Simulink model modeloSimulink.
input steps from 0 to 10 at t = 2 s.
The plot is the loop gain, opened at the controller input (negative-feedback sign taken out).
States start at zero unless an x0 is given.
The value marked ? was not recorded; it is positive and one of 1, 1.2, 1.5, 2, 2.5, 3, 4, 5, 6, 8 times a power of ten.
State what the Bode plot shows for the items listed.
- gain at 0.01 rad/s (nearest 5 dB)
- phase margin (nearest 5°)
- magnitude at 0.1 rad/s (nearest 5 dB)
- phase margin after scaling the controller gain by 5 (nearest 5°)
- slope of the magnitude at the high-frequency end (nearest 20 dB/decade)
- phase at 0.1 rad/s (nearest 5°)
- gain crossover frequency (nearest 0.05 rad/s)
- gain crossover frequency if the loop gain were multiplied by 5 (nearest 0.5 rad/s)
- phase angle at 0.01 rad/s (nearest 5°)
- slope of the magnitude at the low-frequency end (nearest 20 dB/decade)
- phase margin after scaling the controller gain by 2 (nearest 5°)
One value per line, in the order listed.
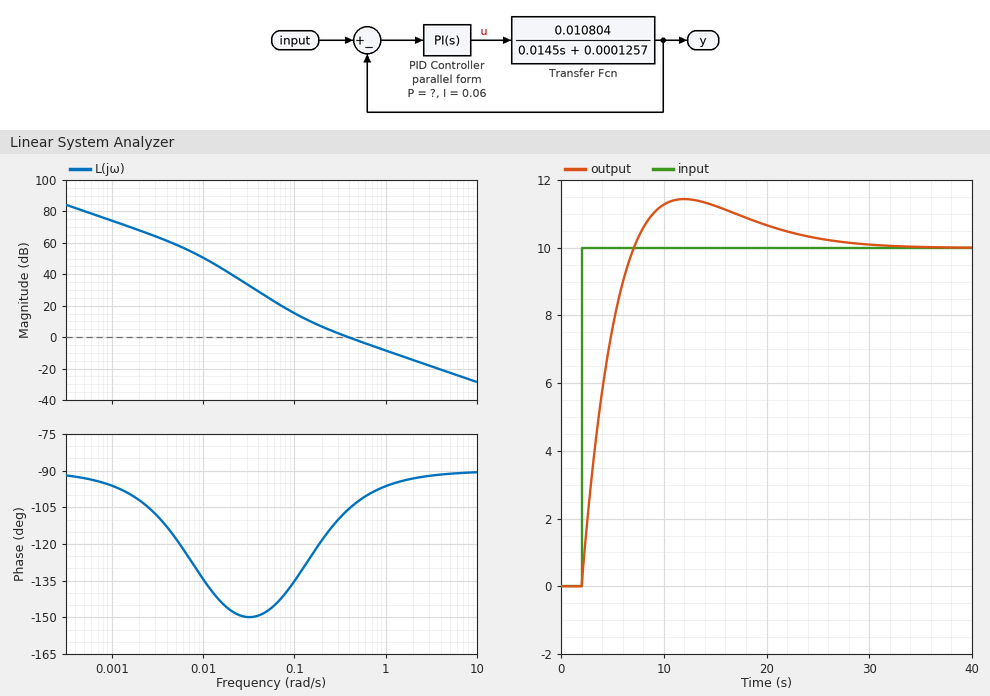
50 dB
75°
15 dB
85°
-20 dB/decade
-135°
0.40 rad/s
2.0 rad/s
-135°
-20 dB/decade
80°
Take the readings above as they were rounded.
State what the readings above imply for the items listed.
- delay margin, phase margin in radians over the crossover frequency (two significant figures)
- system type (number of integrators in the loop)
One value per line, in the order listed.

3.3 s
1
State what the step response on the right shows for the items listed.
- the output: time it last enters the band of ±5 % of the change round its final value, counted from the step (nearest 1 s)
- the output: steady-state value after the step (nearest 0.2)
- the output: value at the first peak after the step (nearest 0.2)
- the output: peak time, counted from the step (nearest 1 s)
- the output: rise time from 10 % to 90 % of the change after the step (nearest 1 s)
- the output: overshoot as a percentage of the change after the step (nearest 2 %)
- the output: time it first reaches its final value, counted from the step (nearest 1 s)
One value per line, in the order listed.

20 s
10.0
11.4
10 s
4 s
14 %
5 s
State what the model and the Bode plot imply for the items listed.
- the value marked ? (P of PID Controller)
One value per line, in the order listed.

0.5
